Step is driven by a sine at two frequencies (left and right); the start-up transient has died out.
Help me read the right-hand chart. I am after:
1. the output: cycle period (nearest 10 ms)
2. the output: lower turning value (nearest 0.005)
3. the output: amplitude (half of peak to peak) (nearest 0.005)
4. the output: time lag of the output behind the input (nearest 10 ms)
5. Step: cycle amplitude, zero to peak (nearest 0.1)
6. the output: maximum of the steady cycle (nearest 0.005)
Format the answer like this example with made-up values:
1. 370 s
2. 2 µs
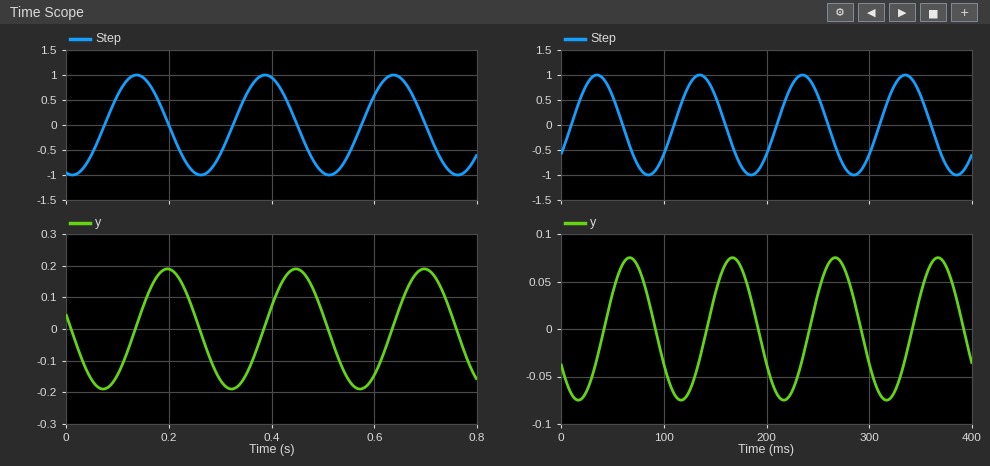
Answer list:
1. 100 ms
2. -0.075
3. 0.075
4. 30 ms
5. 1.0
6. 0.075
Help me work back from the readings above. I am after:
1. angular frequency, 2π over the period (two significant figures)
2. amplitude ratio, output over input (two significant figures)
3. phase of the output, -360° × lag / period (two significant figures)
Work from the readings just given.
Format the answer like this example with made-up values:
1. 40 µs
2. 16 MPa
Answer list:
1. 0.063 rad/ms
2. 0.075
3. -110°
